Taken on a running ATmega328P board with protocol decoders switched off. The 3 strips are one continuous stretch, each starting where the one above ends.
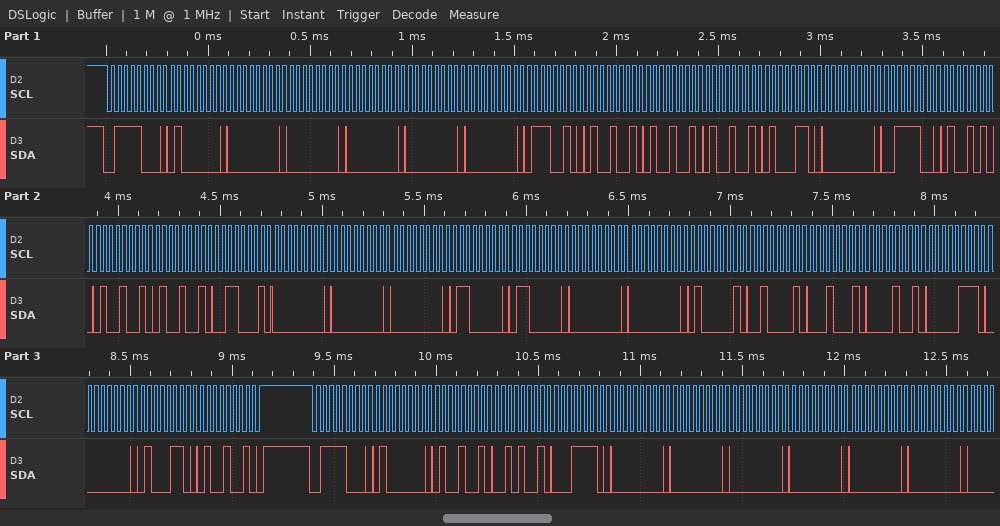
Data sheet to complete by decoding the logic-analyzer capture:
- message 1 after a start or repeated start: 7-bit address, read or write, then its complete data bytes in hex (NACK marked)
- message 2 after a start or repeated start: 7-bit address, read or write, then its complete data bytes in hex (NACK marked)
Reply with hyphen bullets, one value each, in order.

- 0x3C write: 40 00 00 00 00 00 72 49 49 49 46 00 3C 4A 49 49 31 00 00 00 60 60 00 00 41 21 11 09 07 00 46 49
- 0x3C write: 40 49 29 1E 00 00 00 00 00 00
